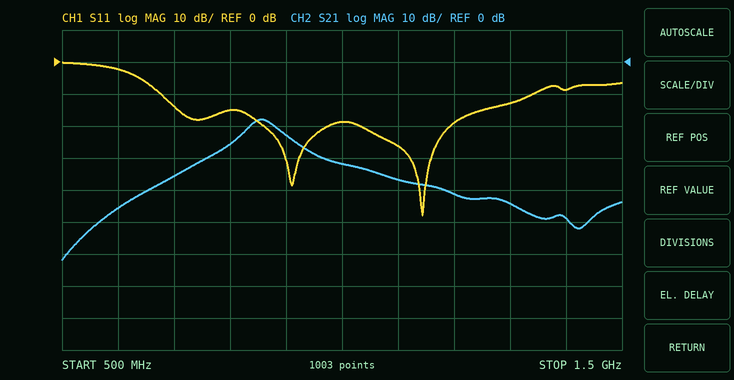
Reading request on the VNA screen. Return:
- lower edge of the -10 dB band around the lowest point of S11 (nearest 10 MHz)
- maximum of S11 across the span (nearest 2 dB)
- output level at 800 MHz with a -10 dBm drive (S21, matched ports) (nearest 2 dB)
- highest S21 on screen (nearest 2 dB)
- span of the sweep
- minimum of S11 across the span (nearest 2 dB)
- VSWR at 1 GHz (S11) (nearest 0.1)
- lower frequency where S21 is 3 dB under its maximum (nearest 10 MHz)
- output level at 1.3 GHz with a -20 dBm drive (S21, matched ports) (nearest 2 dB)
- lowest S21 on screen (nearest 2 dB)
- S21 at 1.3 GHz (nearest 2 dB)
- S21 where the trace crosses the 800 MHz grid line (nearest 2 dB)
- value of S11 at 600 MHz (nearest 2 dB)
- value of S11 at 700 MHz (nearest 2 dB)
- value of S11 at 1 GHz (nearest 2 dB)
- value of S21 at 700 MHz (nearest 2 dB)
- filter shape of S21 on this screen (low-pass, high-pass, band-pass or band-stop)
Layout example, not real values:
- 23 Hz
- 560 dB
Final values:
- 680 MHz
- 0 dB
- -36 dBm
- -18 dB
- 1 GHz
- -48 dB
- 1.3
- 830 MHz
- -64 dBm
- -62 dB
- -44 dB
- -26 dB
- -2 dB
- -14 dB
- -18 dB
- -36 dB
- band-pass
